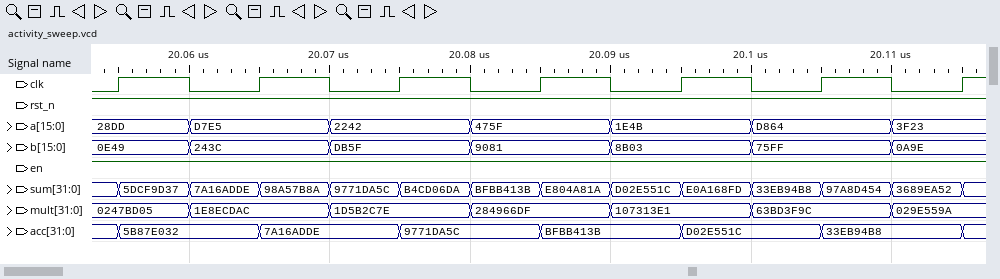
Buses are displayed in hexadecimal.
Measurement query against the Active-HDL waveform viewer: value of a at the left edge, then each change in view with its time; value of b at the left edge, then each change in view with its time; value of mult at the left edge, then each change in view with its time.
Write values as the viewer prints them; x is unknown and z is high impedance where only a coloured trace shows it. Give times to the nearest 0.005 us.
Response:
28DD, D7E5 at 20.06 us, 2242 at 20.07 us, 475F at 20.08 us, 1E4B at 20.09 us, D864 at 20.1 us, 3F23 at 20.11 us
0E49, 243C at 20.06 us, DB5F at 20.07 us, 9081 at 20.08 us, 8B03 at 20.09 us, 75FF at 20.1 us, 0A9E at 20.11 us
0247BD05, 1E8ECDAC at 20.06 us, 1D5B2C7E at 20.07 us, 284966DF at 20.08 us, 107313E1 at 20.09 us, 63BD3F9C at 20.1 us, 029E559A at 20.11 us
